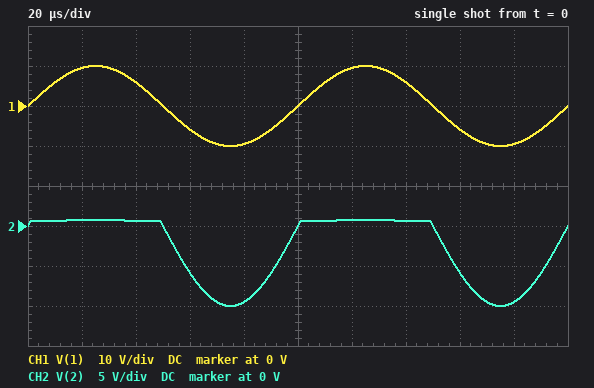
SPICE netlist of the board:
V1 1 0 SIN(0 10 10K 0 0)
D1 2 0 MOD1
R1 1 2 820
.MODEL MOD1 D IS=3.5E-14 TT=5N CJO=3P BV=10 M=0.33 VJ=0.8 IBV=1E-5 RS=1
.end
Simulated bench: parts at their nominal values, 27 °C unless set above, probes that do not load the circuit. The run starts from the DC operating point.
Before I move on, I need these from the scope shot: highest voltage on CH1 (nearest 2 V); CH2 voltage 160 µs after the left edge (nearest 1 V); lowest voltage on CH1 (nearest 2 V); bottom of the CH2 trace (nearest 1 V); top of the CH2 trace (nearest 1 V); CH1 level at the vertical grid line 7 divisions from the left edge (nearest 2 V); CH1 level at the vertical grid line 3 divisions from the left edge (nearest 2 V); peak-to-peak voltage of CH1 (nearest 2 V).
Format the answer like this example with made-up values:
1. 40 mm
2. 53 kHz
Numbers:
1. 10 V
2. -6 V
3. -10 V
4. -10 V
5. 1 V
6. 6 V
7. -6 V
8. 20 V
